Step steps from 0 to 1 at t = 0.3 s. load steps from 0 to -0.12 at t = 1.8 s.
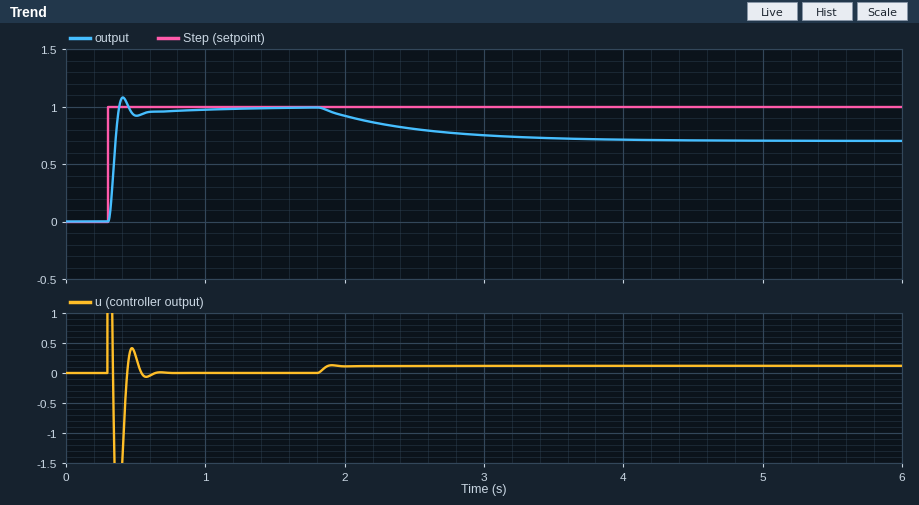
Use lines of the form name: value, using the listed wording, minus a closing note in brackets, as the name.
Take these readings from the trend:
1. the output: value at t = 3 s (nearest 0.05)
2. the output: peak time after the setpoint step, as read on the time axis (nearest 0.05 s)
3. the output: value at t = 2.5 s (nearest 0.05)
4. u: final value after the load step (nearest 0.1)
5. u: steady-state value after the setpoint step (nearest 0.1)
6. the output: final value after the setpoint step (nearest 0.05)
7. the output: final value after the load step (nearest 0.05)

the output: value at t = 3 s: 0.75
the output: peak time after the setpoint step, as read on the time axis: 0.40 s
the output: value at t = 2.5 s: 0.80
u: final value after the load step: 0.1
u: steady-state value after the setpoint step: 0.0
the output: final value after the setpoint step: 1.00
the output: final value after the load step: 0.70
